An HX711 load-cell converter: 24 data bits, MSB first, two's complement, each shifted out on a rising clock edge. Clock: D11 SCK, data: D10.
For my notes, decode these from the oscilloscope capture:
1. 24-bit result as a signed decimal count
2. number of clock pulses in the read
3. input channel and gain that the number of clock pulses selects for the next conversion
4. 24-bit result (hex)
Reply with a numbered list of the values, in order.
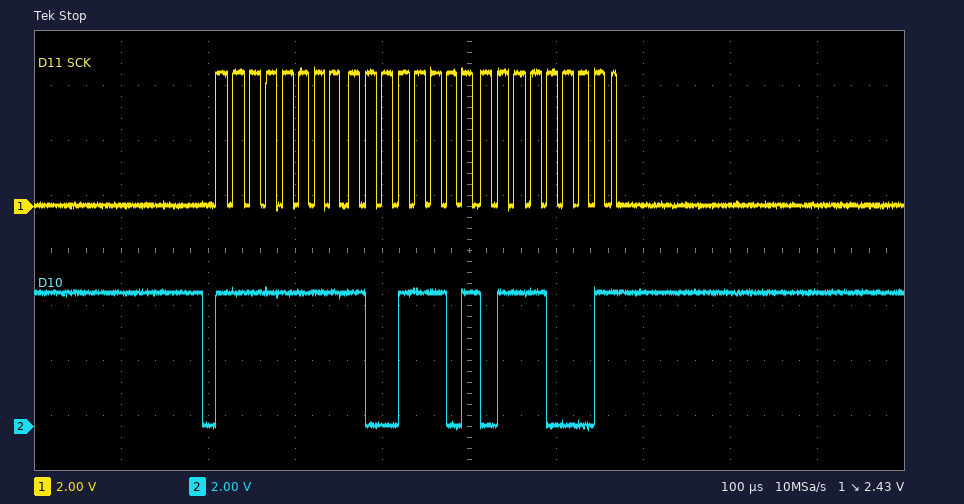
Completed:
1. -25231
2. 25
3. channel A, gain 128
4. 0xFF9D71
